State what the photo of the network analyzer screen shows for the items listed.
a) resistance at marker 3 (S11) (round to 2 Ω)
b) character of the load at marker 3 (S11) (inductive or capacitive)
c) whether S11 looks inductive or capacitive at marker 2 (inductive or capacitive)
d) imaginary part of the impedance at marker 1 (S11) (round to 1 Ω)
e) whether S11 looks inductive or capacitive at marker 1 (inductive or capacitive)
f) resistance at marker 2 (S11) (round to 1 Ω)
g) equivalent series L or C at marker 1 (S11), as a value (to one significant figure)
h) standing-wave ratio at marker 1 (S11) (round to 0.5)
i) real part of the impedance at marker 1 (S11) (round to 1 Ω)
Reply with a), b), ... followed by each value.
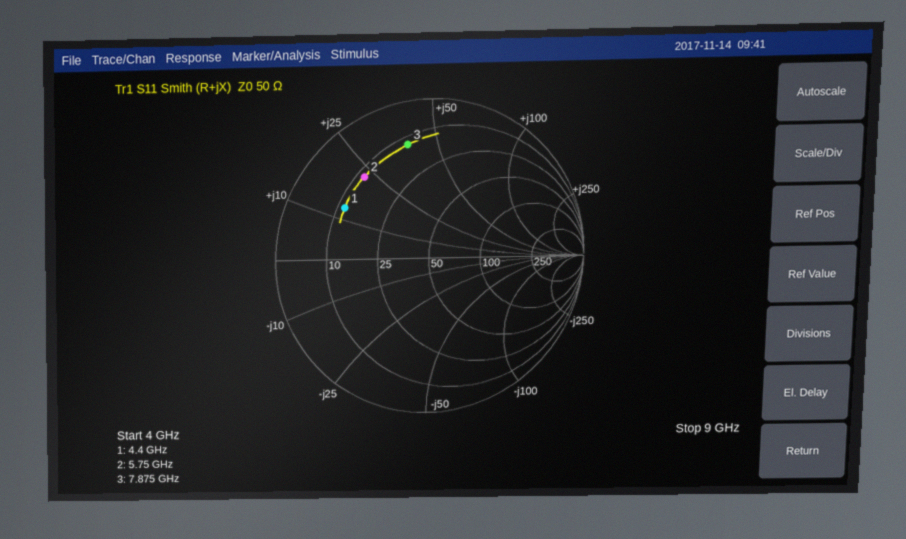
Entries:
a) 12 Ω
b) inductive
c) inductive
d) +13 Ω
e) inductive
f) 12 Ω
g) 500 pH
h) 4.5
i) 12 Ω
